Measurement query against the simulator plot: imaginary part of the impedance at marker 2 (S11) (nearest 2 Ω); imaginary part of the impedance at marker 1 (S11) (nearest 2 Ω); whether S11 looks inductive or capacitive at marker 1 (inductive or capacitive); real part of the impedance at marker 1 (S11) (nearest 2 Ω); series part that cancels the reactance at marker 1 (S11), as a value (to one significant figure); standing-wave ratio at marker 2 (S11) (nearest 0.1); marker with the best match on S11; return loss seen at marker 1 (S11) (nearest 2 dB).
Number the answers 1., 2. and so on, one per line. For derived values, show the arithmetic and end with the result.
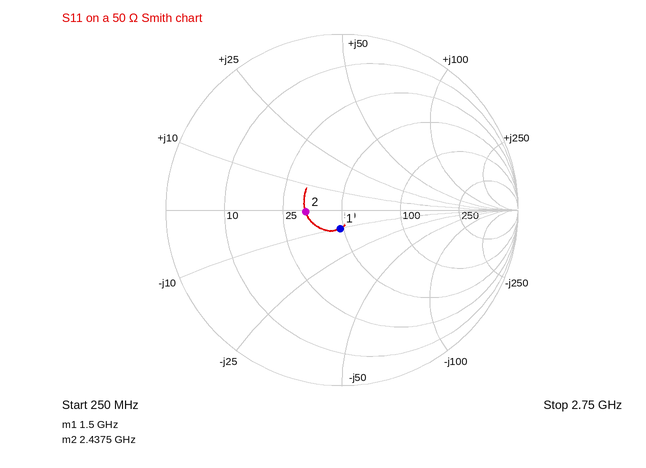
1. 0 Ω
2. -10 Ω
3. capacitive
4. 48 Ω
5. L = 10 Ω/(2π × 1.5 GHz) ≈ 1 nH
6. 1.5
7. marker 1
8. 20 dB
